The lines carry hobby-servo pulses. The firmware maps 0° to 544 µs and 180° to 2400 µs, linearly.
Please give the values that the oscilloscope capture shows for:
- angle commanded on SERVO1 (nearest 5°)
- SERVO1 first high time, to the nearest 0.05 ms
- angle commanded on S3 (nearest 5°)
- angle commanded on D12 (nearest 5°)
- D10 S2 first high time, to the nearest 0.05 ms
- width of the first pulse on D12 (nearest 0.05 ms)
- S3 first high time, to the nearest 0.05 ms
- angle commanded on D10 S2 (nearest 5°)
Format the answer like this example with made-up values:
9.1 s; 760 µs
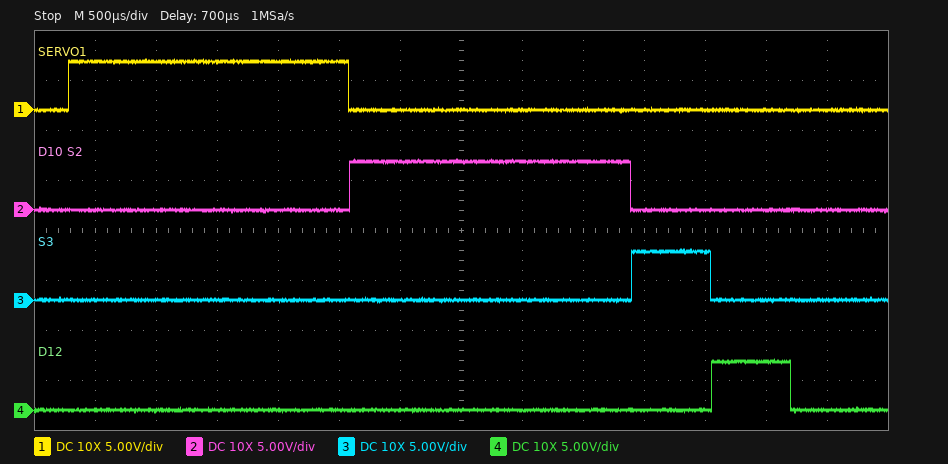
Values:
170°; 2.30 ms; 10°; 10°; 2.30 ms; 0.65 ms; 0.65 ms; 170°
